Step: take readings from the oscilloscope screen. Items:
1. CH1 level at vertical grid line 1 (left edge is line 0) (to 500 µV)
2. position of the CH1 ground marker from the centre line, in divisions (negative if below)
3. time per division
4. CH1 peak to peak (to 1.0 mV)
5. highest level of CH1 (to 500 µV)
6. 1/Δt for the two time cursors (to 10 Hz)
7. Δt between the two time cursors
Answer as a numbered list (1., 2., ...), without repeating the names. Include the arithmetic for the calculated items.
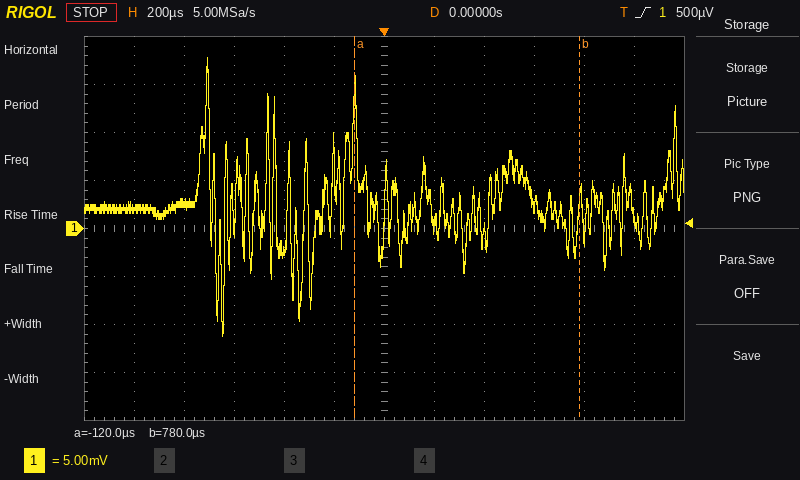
1. 2.0 mV
2. 0.0 div
3. 200 µs
4. 29.0 mV
5. 18.0 mV
6. 1 / 900 µs ≈ 1.11 kHz
7. 780 µs − (-120 µs) = 900 µs
